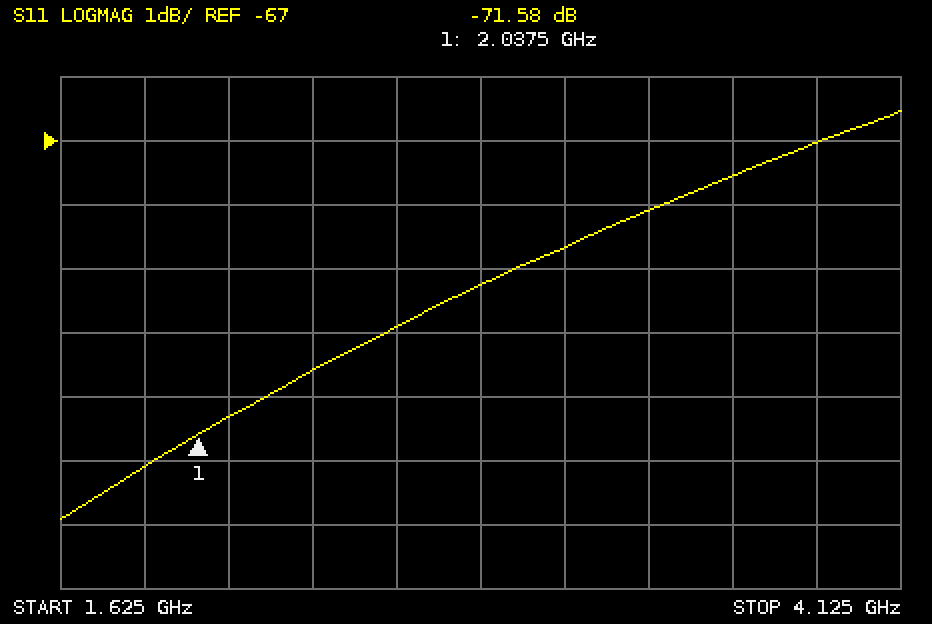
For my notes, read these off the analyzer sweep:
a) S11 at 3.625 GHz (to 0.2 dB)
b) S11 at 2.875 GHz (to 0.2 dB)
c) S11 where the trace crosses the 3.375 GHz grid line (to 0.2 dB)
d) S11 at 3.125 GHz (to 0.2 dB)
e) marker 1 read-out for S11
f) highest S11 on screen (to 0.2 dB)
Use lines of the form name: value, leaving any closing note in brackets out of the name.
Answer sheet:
S11 at 3.625 GHz: -67.6 dB
S11 at 2.875 GHz: -69.2 dB
S11 where the trace crosses the 3.375 GHz grid line: -68.0 dB
S11 at 3.125 GHz: -68.6 dB
marker 1 read-out for S11: -71.58 dB
highest S11 on screen: -66.6 dB
